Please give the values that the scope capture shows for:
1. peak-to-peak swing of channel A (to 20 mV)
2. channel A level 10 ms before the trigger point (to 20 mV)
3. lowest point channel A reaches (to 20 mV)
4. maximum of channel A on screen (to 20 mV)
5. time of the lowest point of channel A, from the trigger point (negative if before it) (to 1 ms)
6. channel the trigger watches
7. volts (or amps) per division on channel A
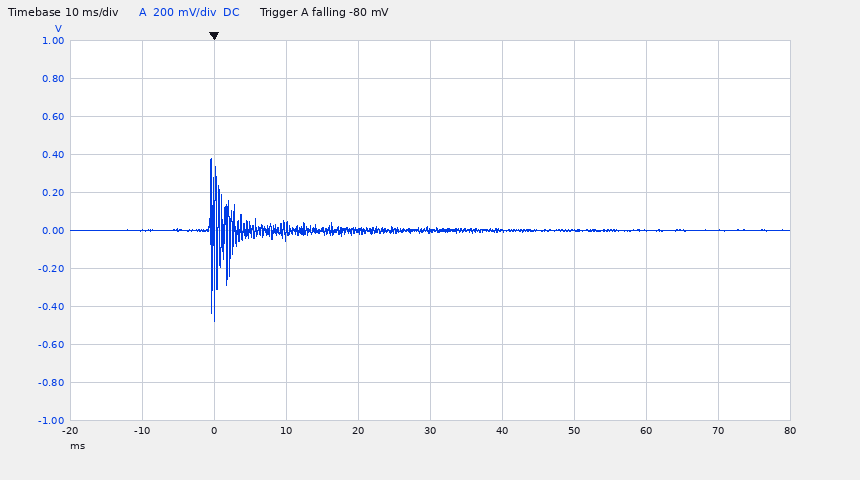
860 mV
0 mV
-480 mV
380 mV
0 ms
channel A
200 mV
